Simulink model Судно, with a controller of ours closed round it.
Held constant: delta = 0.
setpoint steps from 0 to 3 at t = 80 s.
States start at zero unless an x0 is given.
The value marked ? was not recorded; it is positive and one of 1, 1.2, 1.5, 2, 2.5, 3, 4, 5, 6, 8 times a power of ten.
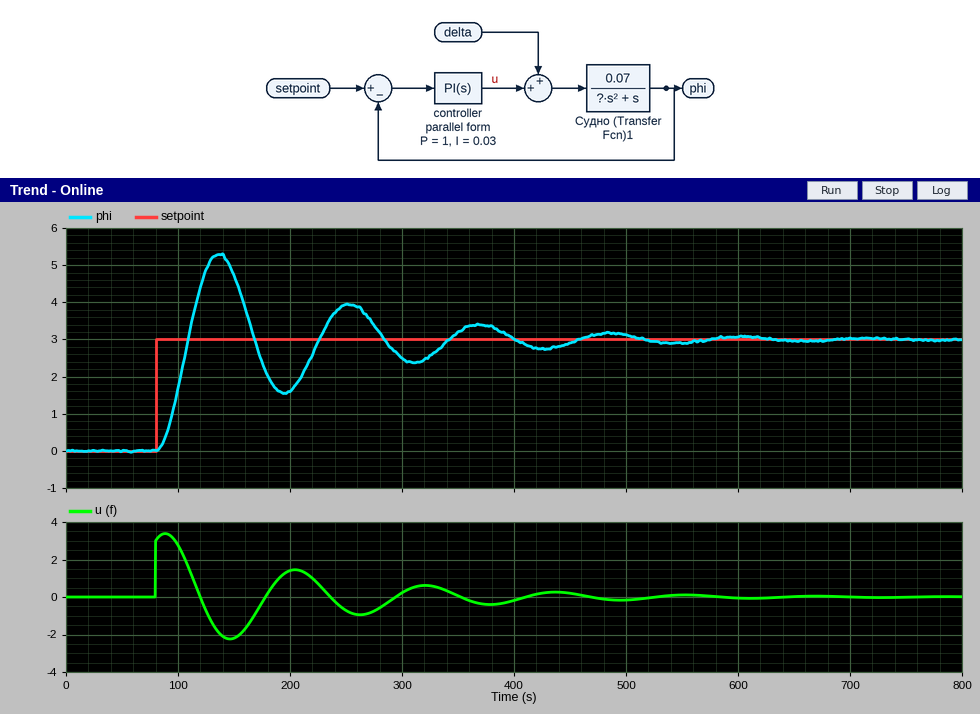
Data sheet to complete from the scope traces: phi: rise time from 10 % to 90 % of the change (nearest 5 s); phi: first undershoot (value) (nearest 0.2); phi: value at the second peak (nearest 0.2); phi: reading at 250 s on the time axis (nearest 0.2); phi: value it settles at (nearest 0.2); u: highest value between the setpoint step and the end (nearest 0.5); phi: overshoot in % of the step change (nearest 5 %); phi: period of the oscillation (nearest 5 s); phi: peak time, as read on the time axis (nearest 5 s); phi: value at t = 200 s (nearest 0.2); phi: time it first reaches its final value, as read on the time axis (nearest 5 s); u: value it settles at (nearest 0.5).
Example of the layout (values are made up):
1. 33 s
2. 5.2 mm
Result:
1. 20 s
2. 1.6
3. 4.0
4. 4.0
5. 3.0
6. 3.5
7. 75 %
8. 115 s
9. 135 s
10. 1.6
11. 110 s
12. 0.0
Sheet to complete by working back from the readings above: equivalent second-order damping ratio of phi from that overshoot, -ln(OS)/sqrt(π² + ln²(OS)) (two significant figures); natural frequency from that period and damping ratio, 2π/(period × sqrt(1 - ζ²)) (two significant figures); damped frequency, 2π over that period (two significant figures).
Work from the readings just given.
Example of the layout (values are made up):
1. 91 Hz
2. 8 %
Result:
1. 0.091
2. 0.055 rad/s
3. 0.055 rad/s
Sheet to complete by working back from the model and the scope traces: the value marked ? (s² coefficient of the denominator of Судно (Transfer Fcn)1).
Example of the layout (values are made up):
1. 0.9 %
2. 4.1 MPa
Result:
1. 20
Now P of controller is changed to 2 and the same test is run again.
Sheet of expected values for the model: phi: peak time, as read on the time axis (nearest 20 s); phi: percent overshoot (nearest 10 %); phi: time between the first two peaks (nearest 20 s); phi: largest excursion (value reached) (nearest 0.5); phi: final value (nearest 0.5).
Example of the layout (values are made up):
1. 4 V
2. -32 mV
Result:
1. 120 s
2. 60 %
3. 80 s
4. 5.0
5. 3.0
